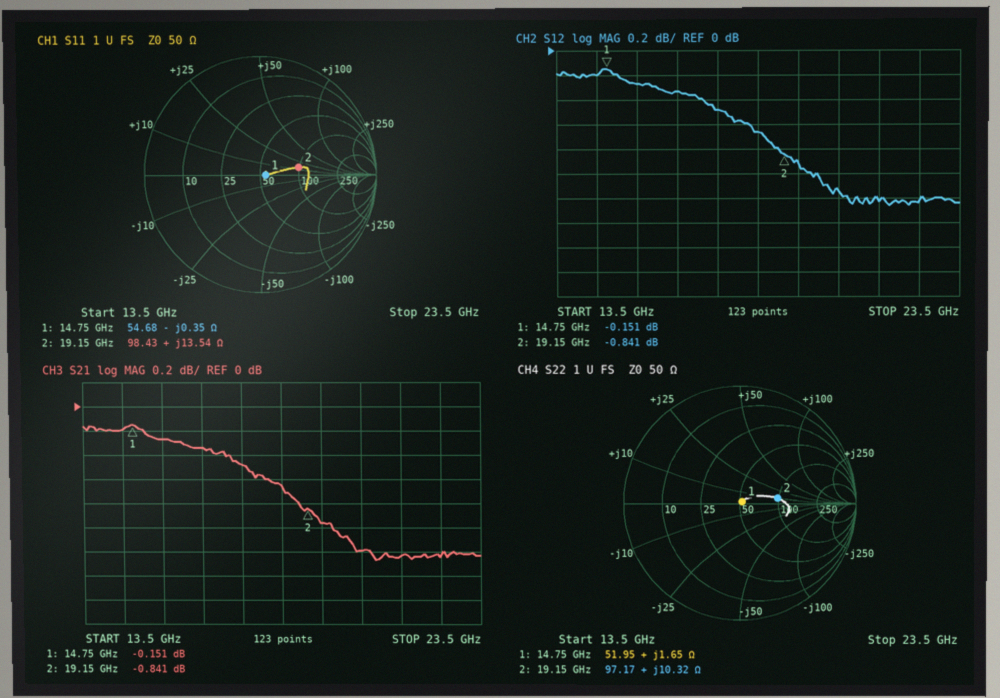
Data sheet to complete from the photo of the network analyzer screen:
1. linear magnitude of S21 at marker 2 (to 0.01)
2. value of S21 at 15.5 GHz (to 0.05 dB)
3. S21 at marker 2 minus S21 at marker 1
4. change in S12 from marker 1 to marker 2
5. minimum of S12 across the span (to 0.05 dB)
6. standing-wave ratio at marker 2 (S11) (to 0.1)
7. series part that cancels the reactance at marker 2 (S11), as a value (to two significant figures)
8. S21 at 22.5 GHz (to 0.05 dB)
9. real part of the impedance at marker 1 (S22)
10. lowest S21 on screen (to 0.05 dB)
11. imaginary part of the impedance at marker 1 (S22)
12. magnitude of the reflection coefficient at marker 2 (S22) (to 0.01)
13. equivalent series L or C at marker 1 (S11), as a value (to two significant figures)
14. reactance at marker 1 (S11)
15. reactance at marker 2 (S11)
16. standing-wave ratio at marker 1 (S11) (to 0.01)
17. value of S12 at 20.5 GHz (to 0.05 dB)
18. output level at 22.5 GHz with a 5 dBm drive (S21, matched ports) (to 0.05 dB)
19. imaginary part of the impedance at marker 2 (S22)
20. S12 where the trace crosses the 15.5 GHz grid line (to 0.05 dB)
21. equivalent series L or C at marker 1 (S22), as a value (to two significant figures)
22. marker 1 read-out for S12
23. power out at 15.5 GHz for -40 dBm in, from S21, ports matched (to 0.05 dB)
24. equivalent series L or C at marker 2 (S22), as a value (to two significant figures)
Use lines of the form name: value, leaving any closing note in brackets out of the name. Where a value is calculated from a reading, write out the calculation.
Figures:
linear magnitude of S21 at marker 2: 10^(-0.841/20) ≈ 0.91
value of S21 at 15.5 GHz: -0.25 dB
S21 at marker 2 minus S21 at marker 1: -0.841 − (-0.151) = -0.690 dB
change in S12 from marker 1 to marker 2: -0.841 − (-0.151) = -0.690 dB
minimum of S12 across the span: -1.25 dB
standing-wave ratio at marker 2 (S11): 2.0
series part that cancels the reactance at marker 2 (S11), as a value: C = 1/(2π × 19.15 GHz × 13.54 Ω) ≈ 614 fF, so 610 fF to two significant figures
S21 at 22.5 GHz: -1.25 dB
real part of the impedance at marker 1: 51.95 Ω
lowest S21 on screen: -1.25 dB
imaginary part of the impedance at marker 1: +1.65 Ω
magnitude of the reflection coefficient at marker 2 (S22): 0.33
equivalent series L or C at marker 1 (S11), as a value: C = 1/(2π × 14.75 GHz × 0.35 Ω) ≈ 31 pF
reactance at marker 1: -0.35 Ω
reactance at marker 2: +13.54 Ω
standing-wave ratio at marker 1 (S11): 1.09
value of S12 at 20.5 GHz: -1.15 dB
output level at 22.5 GHz with a 5 dBm drive (S21, matched ports): 5 dBm + (-1.25 dB) = 3.75 dBm
imaginary part of the impedance at marker 2: +10.32 Ω
S12 where the trace crosses the 15.5 GHz grid line: -0.25 dB
equivalent series L or C at marker 1 (S22), as a value: L = 1.65 Ω/(2π × 14.75 GHz) ≈ 18 pH
marker 1 read-out for S12: -0.151 dB
power out at 15.5 GHz for -40 dBm in, from S21, ports matched: -40 dBm + (-0.25 dB) = -40.25 dBm
equivalent series L or C at marker 2 (S22), as a value: L = 10.32 Ω/(2π × 19.15 GHz) ≈ 86 pH
